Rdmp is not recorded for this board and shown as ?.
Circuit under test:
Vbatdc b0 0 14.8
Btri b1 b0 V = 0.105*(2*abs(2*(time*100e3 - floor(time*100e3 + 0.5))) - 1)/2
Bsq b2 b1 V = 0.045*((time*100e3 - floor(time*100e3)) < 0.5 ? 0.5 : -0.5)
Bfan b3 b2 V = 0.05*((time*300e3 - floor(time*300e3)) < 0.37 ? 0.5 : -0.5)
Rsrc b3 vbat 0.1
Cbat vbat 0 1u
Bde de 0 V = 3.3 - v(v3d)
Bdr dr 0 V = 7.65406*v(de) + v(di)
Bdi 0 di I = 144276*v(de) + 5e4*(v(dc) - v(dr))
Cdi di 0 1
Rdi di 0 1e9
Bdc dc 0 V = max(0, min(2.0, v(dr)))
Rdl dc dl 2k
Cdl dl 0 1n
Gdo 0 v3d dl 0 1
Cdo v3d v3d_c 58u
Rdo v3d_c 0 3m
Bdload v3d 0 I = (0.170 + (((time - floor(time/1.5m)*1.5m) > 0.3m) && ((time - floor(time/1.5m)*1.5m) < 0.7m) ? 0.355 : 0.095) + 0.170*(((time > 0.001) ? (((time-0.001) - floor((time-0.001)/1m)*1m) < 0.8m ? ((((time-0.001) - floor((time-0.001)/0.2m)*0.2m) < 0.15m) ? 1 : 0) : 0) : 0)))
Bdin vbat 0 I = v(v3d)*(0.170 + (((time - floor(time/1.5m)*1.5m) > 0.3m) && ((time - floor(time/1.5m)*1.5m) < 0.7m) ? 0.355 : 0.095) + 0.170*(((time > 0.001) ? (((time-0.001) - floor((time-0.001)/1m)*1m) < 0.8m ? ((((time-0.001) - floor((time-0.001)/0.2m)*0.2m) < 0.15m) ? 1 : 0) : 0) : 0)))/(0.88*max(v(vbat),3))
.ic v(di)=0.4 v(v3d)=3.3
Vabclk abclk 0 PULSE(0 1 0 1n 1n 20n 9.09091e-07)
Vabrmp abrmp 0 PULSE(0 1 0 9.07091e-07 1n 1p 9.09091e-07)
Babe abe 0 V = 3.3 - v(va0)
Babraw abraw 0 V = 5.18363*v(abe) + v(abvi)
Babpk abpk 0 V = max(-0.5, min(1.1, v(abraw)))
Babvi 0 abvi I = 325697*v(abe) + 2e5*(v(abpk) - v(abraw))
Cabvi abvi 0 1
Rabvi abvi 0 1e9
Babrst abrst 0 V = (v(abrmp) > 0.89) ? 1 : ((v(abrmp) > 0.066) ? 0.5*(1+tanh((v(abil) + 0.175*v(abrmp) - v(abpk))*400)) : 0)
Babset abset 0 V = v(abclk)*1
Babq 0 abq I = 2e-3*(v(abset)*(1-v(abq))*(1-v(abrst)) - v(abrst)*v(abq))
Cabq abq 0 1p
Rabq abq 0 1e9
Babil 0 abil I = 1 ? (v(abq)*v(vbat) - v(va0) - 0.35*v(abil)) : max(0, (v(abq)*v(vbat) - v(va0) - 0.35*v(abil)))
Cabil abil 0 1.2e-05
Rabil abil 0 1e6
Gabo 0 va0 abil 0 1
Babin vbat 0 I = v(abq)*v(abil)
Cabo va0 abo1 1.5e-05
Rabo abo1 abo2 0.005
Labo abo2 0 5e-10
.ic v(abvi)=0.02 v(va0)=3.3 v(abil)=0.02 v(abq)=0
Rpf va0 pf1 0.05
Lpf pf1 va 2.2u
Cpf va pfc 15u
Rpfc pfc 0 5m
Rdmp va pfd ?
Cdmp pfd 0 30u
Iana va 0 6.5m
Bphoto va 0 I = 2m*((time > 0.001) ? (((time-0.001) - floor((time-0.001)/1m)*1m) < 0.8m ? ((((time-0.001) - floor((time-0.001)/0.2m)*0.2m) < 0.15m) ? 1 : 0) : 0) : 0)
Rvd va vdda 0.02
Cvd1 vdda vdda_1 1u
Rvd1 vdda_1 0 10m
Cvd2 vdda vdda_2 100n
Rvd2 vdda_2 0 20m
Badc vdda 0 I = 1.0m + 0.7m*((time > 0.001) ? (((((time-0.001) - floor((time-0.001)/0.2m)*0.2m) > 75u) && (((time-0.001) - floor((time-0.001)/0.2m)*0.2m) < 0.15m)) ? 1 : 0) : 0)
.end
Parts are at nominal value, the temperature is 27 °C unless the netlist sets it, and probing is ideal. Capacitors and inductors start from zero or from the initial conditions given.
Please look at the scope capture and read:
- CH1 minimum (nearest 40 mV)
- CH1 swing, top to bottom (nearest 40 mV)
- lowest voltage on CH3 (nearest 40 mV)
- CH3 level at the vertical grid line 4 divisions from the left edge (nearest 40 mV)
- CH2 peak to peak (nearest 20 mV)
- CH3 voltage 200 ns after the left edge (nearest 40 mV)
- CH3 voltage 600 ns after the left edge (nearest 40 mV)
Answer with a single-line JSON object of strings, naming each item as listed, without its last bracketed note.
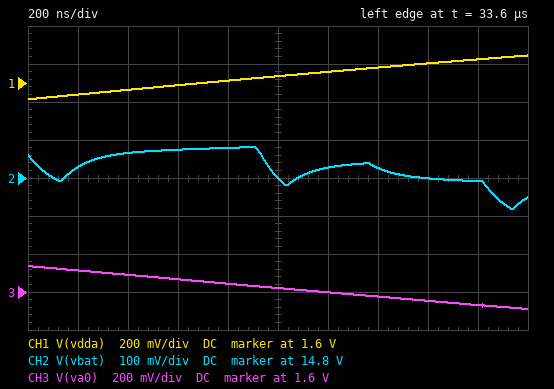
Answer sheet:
{"CH1 minimum": "1.52 V", "CH1 swing, top to bottom": "240 mV", "lowest voltage on CH3": "1.52 V", "CH3 level at the vertical grid line 4 divisions from the left edge": "1.64 V", "CH2 peak to peak": "160 mV", "CH3 voltage 200 ns after the left edge": "1.72 V", "CH3 voltage 600 ns after the left edge": "1.68 V"}
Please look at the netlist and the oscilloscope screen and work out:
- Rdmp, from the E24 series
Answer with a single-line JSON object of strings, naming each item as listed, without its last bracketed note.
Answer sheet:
{"Rdmp, from the E24 series": "0.68 Ω"}
